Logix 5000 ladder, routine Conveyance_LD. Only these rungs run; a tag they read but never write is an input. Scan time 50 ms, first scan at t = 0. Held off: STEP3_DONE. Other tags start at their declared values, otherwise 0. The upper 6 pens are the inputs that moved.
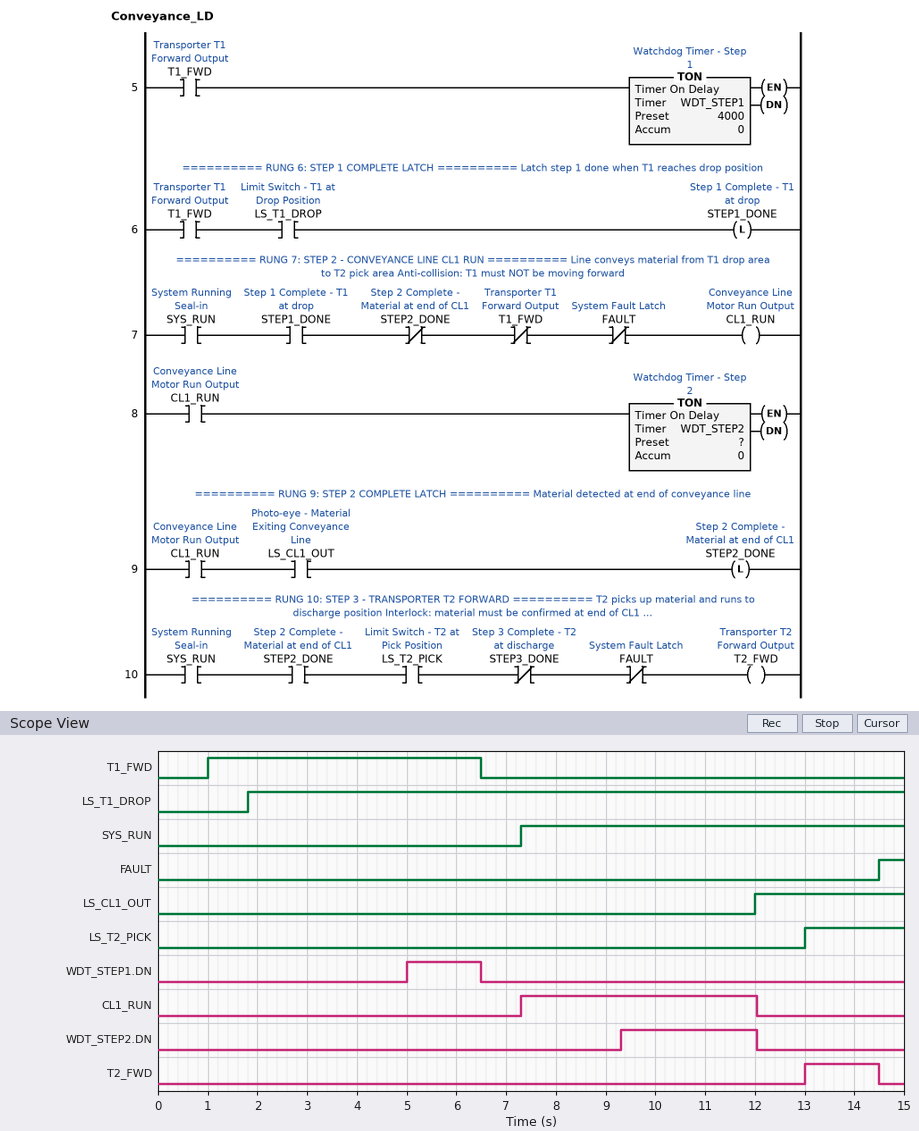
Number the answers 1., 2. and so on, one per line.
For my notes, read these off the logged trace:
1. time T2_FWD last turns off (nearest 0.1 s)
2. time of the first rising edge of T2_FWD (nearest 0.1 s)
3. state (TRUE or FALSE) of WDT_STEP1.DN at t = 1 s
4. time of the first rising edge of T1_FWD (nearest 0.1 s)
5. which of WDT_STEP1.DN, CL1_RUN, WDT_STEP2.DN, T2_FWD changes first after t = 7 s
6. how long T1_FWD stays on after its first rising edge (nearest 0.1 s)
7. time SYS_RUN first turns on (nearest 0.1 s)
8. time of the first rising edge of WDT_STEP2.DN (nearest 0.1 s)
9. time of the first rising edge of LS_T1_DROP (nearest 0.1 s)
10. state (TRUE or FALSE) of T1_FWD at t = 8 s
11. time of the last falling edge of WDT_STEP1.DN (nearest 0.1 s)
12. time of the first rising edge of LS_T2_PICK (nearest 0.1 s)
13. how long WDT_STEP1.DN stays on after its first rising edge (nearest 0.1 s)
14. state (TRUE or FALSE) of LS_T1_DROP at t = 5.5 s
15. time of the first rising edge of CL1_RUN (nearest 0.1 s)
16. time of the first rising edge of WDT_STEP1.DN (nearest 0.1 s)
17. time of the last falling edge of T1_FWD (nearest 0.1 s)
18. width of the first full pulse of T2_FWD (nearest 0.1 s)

1. 14.5 s
2. 13.0 s
3. FALSE
4. 1.0 s
5. CL1_RUN
6. 5.5 s
7. 7.3 s
8. 9.3 s
9. 1.8 s
10. FALSE
11. 6.5 s
12. 13.0 s
13. 1.5 s
14. TRUE
15. 7.3 s
16. 5.0 s
17. 6.5 s
18. 1.5 s
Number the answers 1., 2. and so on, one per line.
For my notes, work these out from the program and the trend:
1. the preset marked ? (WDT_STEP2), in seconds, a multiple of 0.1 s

1. 2.0 s
